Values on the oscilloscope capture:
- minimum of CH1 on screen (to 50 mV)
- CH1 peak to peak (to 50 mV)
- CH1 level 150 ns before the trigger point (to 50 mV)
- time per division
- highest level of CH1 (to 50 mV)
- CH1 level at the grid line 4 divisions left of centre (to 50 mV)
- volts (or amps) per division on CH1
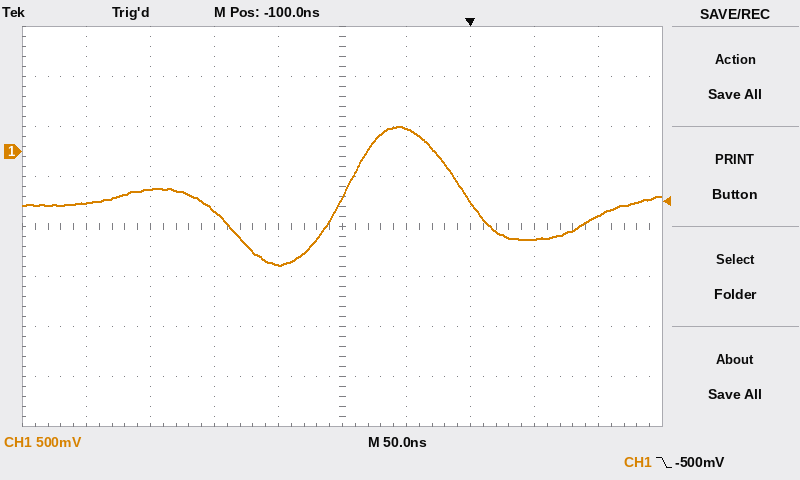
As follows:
-1.15 V
1.40 V
-1.15 V
50 ns
250 mV
-500 mV
500 mV
